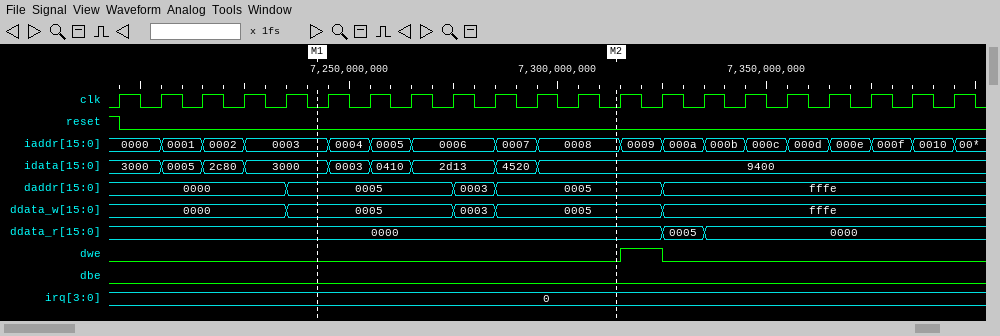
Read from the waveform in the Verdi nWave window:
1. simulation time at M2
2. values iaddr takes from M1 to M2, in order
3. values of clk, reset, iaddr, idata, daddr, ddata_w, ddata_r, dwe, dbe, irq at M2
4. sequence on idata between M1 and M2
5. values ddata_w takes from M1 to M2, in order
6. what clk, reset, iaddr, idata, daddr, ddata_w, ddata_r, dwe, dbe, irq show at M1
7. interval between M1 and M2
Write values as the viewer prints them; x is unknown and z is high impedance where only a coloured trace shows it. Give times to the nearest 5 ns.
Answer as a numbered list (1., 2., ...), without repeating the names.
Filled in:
1. 7315 ns
2. 0003, 0004, 0005, 0006, 0007, 0008
3. clk=0, reset=0, iaddr=0008, idata=9400, daddr=0005, ddata_w=0005, ddata_r=0000, dwe=0, dbe=0, irq=0
4. 3000, 0003, 0410, 2d13, 4520, 9400
5. 0005, 0003, 0005
6. clk=0, reset=0, iaddr=0003, idata=3000, daddr=0005, ddata_w=0005, ddata_r=0000, dwe=0, dbe=0, irq=0
7. 70 ns
